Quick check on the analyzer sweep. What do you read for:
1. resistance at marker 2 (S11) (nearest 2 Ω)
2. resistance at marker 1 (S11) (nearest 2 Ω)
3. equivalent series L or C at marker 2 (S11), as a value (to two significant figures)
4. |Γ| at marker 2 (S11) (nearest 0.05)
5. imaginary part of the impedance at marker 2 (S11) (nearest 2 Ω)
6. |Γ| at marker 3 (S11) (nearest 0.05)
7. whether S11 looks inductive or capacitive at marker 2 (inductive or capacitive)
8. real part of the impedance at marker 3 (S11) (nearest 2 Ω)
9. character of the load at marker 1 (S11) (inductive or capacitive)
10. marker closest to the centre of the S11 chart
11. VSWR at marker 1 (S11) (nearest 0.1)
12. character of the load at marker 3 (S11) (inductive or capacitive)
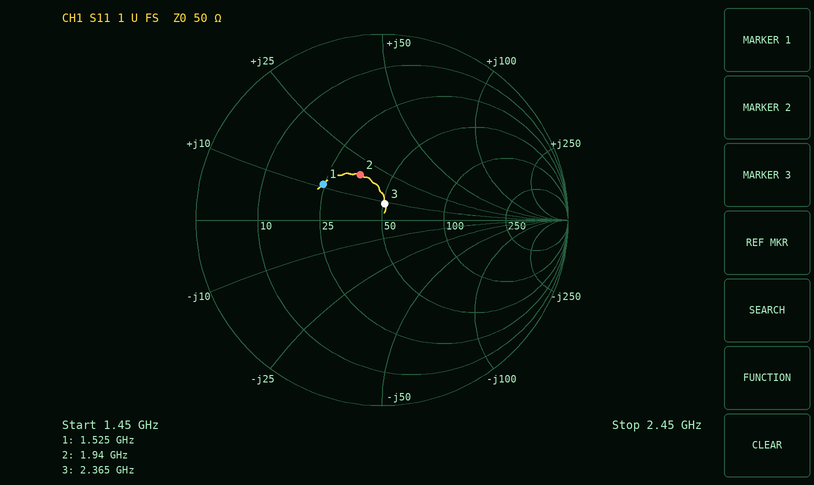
36 Ω
24 Ω
1.5 nH
0.25
+18 Ω
0.10
inductive
50 Ω
inductive
marker 3
2.2
inductive
